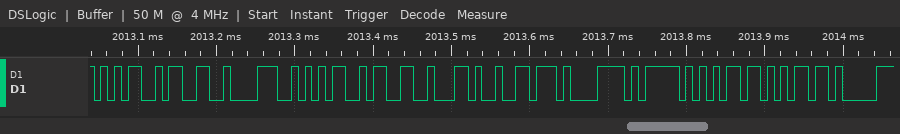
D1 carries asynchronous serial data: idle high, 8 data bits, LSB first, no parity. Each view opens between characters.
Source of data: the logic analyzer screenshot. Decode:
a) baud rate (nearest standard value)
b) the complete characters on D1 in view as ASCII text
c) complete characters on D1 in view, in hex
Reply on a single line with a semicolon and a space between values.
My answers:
115200 baud; "53853,vx_mm"; 35, 33, 38, 35, 33, 2C, 76, 78, 5F, 6D, 6D
